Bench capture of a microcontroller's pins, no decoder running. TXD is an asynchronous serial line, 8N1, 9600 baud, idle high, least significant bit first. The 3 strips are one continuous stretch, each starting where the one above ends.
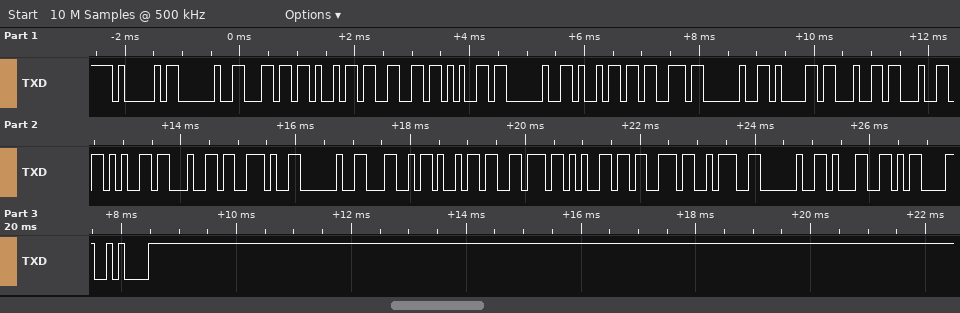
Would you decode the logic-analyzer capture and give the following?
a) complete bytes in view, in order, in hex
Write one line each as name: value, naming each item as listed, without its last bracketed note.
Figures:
complete bytes in view, in order, in hex: 41 20 6C 69 66 65 20 69 73 20 61 64 64 65 64 2E 20 4C 69 76 65 73 3A 20 31 0D 0A
